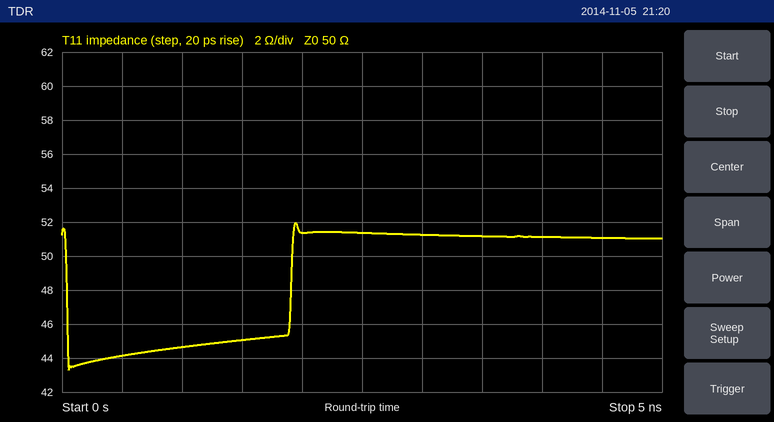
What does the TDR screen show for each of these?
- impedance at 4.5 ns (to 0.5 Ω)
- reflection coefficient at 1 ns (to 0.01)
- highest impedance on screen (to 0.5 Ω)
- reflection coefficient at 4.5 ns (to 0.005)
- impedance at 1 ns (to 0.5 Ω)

51.0 Ω
-0.06
52.0 Ω
+0.010
44.5 Ω
